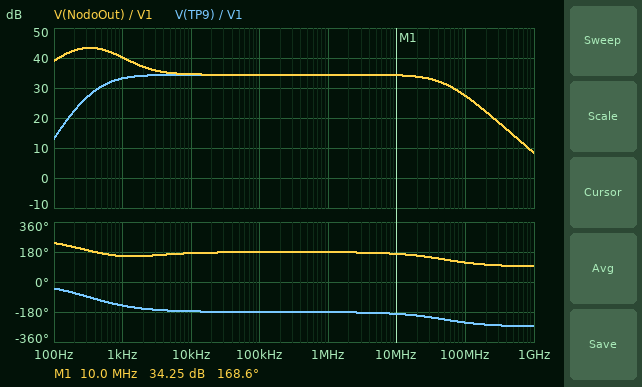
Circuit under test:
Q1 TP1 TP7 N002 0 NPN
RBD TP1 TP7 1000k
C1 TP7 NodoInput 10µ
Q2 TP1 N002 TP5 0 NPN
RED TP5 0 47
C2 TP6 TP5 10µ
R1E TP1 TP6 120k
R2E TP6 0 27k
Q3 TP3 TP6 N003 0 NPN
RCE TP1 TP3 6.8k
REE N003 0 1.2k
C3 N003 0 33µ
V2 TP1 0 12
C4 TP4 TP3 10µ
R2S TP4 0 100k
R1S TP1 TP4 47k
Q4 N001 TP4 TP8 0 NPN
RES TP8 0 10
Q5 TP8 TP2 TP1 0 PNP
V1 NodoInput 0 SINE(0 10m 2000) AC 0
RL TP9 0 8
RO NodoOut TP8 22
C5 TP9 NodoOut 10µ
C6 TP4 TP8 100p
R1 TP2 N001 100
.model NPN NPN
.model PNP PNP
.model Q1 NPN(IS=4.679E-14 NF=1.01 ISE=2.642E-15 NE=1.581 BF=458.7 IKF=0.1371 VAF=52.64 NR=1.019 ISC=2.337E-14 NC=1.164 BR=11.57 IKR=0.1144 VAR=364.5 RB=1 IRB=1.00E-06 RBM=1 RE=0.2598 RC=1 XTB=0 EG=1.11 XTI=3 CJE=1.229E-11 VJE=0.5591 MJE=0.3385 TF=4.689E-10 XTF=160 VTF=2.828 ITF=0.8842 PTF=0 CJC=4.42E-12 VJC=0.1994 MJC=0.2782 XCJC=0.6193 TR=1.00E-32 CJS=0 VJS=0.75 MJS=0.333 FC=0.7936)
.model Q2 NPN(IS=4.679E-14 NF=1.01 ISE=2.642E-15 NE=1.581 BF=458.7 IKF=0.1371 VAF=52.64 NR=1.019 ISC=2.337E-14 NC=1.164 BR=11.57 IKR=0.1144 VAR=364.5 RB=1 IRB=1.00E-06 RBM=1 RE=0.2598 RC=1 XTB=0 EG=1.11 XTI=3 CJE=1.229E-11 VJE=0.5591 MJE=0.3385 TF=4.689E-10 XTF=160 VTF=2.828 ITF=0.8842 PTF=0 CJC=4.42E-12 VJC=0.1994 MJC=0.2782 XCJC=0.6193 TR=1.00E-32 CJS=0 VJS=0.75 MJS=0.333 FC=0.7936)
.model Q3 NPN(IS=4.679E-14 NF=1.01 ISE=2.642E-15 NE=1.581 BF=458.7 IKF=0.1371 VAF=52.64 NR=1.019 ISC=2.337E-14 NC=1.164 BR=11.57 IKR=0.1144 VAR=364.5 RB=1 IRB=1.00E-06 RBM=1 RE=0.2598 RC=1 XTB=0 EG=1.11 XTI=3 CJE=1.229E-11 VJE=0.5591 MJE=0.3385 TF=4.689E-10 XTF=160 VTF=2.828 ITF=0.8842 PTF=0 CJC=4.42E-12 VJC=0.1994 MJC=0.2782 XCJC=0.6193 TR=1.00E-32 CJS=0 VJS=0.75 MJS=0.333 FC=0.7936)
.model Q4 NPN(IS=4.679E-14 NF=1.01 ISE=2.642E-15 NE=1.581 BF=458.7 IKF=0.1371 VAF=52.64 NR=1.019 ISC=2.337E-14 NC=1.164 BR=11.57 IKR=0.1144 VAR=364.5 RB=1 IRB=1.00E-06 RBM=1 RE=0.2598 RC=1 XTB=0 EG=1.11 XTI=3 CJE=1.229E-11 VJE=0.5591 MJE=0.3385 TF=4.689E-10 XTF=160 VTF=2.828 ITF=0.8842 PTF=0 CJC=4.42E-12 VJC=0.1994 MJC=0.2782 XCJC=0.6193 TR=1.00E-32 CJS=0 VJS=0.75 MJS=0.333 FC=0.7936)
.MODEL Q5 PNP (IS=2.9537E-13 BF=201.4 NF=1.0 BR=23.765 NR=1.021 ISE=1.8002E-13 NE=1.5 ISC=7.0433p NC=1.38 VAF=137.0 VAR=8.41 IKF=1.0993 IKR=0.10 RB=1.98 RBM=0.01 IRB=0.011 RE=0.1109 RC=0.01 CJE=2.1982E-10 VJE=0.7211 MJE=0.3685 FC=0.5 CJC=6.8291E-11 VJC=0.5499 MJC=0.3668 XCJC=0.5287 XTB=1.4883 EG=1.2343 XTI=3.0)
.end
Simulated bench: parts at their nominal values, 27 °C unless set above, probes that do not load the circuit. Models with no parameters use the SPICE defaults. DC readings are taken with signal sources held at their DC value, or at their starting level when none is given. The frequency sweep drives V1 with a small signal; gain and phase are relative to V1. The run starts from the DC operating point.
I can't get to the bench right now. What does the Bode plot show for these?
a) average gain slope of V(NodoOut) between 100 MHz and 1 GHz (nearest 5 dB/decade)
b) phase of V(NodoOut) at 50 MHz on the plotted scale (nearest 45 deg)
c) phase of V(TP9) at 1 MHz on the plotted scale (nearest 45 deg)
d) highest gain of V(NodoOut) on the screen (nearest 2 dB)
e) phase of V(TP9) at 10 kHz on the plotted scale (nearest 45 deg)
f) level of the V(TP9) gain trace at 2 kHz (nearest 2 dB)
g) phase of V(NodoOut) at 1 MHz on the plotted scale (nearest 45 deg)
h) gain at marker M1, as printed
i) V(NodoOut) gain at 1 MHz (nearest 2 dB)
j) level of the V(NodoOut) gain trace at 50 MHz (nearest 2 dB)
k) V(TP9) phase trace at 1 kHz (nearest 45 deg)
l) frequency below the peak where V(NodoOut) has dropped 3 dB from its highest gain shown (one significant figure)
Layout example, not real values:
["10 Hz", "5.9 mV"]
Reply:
["-20 dB/decade", "135 deg", "-180 deg", "44 dB", "-180 deg", "34 dB", "180 deg", "34.25 dB", "34 dB", "32 dB", "-135 deg", "100 Hz"]
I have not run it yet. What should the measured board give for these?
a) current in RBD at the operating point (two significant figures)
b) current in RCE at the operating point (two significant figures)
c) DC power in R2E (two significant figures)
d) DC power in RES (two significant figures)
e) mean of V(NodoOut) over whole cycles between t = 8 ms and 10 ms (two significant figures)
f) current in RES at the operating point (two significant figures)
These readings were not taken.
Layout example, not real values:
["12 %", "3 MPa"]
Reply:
["7.0 µA", "1.0 mA", "150 µW", "3.1 W", "5.6 V", "560 mA"]
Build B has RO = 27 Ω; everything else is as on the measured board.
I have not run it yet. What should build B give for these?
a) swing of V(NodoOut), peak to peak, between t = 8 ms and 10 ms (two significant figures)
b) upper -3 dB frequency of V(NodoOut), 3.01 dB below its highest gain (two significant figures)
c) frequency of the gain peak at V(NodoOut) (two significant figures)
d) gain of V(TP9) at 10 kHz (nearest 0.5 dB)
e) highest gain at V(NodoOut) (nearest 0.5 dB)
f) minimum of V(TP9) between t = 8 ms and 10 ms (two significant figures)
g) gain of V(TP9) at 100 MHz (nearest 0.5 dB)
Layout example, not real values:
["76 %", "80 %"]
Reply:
["1.2 V", "840 Hz", "310 Hz", "33.0 dB", "43.0 dB", "-470 mV", "26.5 dB"]
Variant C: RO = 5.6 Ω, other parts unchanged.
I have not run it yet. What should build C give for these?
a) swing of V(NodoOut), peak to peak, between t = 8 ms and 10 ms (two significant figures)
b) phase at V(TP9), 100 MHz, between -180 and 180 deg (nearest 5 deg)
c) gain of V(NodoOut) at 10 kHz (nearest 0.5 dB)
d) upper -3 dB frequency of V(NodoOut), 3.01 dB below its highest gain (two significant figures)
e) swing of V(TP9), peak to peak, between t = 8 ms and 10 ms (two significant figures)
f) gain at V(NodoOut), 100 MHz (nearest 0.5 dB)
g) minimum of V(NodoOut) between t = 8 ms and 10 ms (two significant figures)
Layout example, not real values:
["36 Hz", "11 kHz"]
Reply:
["2.7 V", "110 deg", "41.0 dB", "3.4 kHz", "2.0 V", "32.5 dB", "4.1 V"]
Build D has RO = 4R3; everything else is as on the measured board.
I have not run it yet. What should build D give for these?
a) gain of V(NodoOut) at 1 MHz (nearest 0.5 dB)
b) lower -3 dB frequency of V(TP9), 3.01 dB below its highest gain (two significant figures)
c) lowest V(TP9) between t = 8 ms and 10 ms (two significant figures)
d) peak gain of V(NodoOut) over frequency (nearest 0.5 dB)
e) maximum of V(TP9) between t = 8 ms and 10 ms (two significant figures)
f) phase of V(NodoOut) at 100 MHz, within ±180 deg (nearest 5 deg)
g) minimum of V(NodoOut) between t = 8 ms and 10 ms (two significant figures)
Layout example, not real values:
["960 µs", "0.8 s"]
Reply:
["42.0 dB", "1.3 kHz", "-1.1 V", "45.0 dB", "970 mV", "110 deg", "4.0 V"]
